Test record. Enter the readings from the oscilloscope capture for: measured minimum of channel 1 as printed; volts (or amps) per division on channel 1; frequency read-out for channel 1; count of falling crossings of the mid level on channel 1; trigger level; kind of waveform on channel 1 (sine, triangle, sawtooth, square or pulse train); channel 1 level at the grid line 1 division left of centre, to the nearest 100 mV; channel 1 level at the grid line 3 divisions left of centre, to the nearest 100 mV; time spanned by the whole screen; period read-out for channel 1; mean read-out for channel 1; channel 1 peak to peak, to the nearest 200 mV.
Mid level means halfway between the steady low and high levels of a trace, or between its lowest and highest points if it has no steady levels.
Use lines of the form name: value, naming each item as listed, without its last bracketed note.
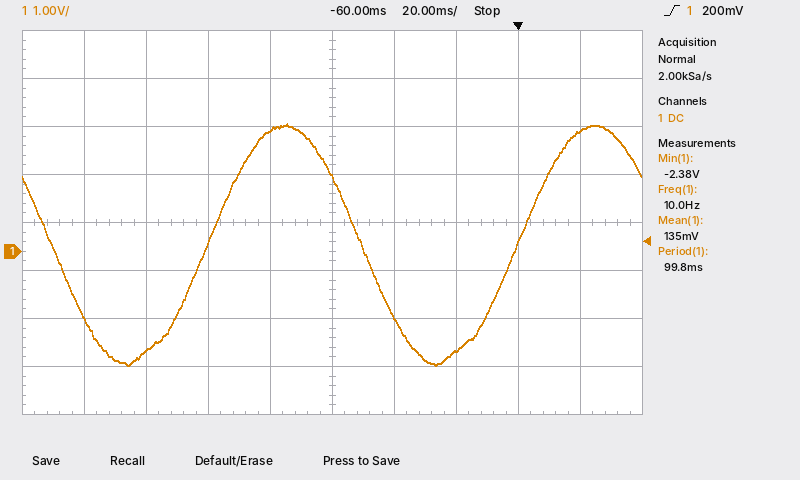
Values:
measured minimum of channel 1 as printed: -2.38 V
volts (or amps) per division on channel 1: 1 V
frequency read-out for channel 1: 10.0 Hz
count of falling crossings of the mid level on channel 1: 2
trigger level: 200 mV
kind of waveform on channel 1: sine
channel 1 level at the grid line 1 division left of centre, to the nearest 100 mV: 2.5 V
channel 1 level at the grid line 3 divisions left of centre, to the nearest 100 mV: -2.1 V
time spanned by the whole screen: 200 ms
period read-out for channel 1: 99.8 ms
mean read-out for channel 1: 135 mV
channel 1 peak to peak, to the nearest 200 mV: 5.0 V
